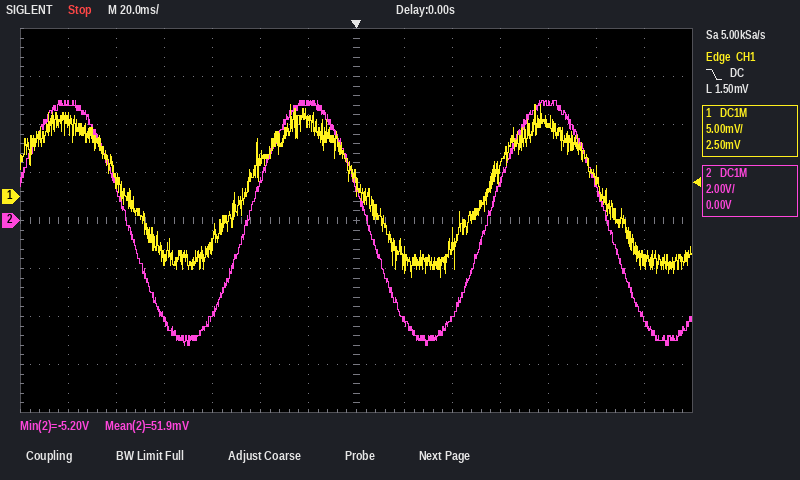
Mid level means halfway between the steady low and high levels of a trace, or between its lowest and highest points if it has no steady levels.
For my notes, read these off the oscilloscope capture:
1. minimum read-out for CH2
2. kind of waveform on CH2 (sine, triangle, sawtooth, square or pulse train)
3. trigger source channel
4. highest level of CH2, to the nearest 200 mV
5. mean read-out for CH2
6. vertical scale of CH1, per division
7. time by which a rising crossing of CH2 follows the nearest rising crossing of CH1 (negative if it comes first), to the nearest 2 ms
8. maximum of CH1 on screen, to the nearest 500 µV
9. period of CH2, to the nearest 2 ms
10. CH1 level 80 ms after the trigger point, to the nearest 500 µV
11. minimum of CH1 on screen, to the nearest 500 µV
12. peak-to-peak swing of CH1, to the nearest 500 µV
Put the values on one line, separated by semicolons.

-5.20 V; sine; CH1; 5.0 V; 51.9 mV; 5 mV; 0 ms; 9.5 mV; 100 ms; 7.5 mV; -8.5 mV; 18.0 mV
